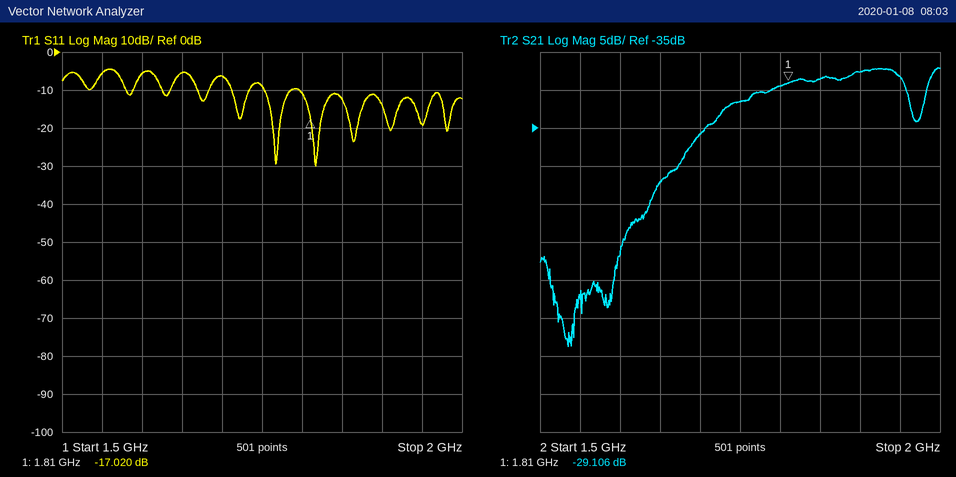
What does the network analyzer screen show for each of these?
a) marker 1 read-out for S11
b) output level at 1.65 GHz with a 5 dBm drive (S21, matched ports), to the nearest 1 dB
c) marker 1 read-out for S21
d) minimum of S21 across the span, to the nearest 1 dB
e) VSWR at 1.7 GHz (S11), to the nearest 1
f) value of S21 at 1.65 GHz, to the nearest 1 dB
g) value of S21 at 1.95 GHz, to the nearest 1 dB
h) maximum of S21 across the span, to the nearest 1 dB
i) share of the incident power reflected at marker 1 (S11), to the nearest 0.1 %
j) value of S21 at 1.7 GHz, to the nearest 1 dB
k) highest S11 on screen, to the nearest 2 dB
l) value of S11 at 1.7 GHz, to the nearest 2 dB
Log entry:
-17.020 dB
-37 dBm
-29.106 dB
-64 dB
3
-42 dB
-28 dB
-27 dB
2.0 %
-36 dB
-4 dB
-6 dB
